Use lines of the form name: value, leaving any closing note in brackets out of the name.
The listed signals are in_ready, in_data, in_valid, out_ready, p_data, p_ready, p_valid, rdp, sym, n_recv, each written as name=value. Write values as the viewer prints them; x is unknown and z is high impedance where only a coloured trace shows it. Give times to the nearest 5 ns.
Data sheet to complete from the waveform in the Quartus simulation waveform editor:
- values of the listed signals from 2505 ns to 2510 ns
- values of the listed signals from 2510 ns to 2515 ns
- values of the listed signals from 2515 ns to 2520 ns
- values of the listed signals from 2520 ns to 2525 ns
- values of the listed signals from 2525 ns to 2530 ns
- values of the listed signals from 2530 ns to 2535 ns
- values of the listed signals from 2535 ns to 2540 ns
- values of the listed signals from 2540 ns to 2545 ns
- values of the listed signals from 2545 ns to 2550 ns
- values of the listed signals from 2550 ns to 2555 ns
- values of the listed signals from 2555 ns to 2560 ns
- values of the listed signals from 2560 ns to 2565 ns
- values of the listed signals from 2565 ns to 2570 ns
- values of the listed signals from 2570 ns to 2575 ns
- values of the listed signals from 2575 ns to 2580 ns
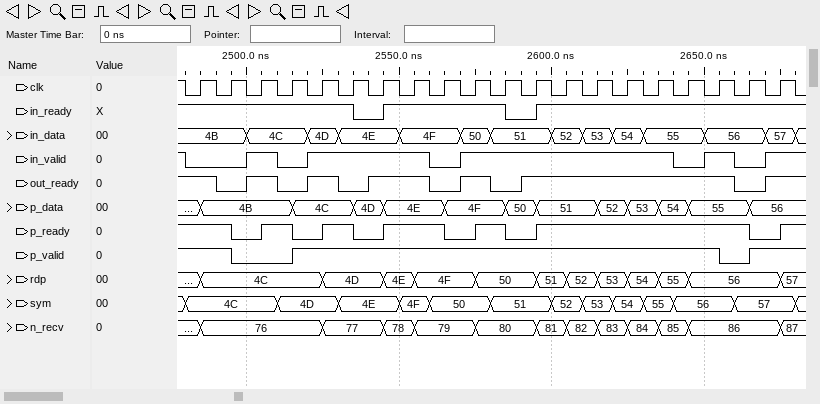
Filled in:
values of the listed signals from 2505 ns to 2510 ns: in_ready=1, in_data=4C, in_valid=1, out_ready=1, p_data=4B, p_ready=1, p_valid=0, rdp=4C, sym=4C, n_recv=76
values of the listed signals from 2510 ns to 2515 ns: in_ready=1, in_data=4C, in_valid=0, out_ready=0, p_data=4B, p_ready=1, p_valid=0, rdp=4C, sym=4D, n_recv=76
values of the listed signals from 2515 ns to 2520 ns: in_ready=1, in_data=4C, in_valid=0, out_ready=0, p_data=4C, p_ready=0, p_valid=1, rdp=4C, sym=4D, n_recv=76
values of the listed signals from 2520 ns to 2525 ns: in_ready=1, in_data=4D, in_valid=1, out_ready=1, p_data=4C, p_ready=0, p_valid=1, rdp=4C, sym=4D, n_recv=76
values of the listed signals from 2525 ns to 2530 ns: in_ready=1, in_data=4D, in_valid=1, out_ready=1, p_data=4C, p_ready=1, p_valid=1, rdp=4D, sym=4D, n_recv=77
values of the listed signals from 2530 ns to 2535 ns: in_ready=1, in_data=4E, in_valid=1, out_ready=0, p_data=4C, p_ready=1, p_valid=1, rdp=4D, sym=4E, n_recv=77
values of the listed signals from 2535 ns to 2540 ns: in_ready=0, in_data=4E, in_valid=1, out_ready=0, p_data=4D, p_ready=0, p_valid=1, rdp=4D, sym=4E, n_recv=77
values of the listed signals from 2540 ns to 2545 ns: in_ready=0, in_data=4E, in_valid=1, out_ready=1, p_data=4D, p_ready=0, p_valid=1, rdp=4D, sym=4E, n_recv=77
values of the listed signals from 2545 ns to 2550 ns: in_ready=1, in_data=4E, in_valid=1, out_ready=1, p_data=4E, p_ready=1, p_valid=1, rdp=4E, sym=4E, n_recv=78
values of the listed signals from 2550 ns to 2555 ns: in_ready=1, in_data=4F, in_valid=1, out_ready=1, p_data=4E, p_ready=1, p_valid=1, rdp=4E, sym=4F, n_recv=78
values of the listed signals from 2555 ns to 2560 ns: in_ready=1, in_data=4F, in_valid=1, out_ready=1, p_data=4E, p_ready=1, p_valid=1, rdp=4F, sym=4F, n_recv=79
values of the listed signals from 2560 ns to 2565 ns: in_ready=1, in_data=4F, in_valid=0, out_ready=0, p_data=4E, p_ready=1, p_valid=1, rdp=4F, sym=50, n_recv=79
values of the listed signals from 2565 ns to 2570 ns: in_ready=1, in_data=4F, in_valid=0, out_ready=0, p_data=4F, p_ready=0, p_valid=1, rdp=4F, sym=50, n_recv=79
values of the listed signals from 2570 ns to 2575 ns: in_ready=1, in_data=50, in_valid=1, out_ready=1, p_data=4F, p_ready=0, p_valid=1, rdp=4F, sym=50, n_recv=79
values of the listed signals from 2575 ns to 2580 ns: in_ready=1, in_data=50, in_valid=1, out_ready=1, p_data=4F, p_ready=1, p_valid=1, rdp=50, sym=50, n_recv=80
